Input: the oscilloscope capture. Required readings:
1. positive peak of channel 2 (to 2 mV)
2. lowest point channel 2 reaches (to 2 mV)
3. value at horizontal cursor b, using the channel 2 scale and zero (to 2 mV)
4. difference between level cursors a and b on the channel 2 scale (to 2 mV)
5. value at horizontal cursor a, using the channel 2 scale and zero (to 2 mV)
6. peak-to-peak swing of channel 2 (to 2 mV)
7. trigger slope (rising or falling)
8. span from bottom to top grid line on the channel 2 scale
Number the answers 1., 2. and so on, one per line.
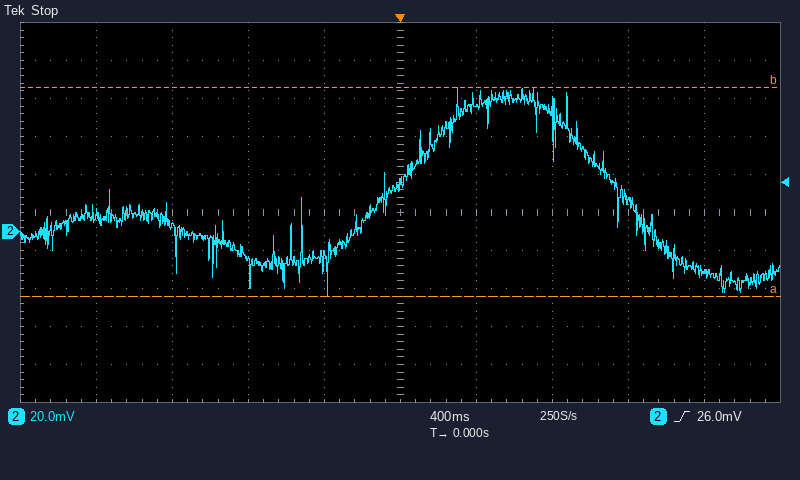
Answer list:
1. 76 mV
2. -34 mV
3. 76 mV
4. 110 mV
5. -34 mV
6. 110 mV
7. rising
8. 200 mV
